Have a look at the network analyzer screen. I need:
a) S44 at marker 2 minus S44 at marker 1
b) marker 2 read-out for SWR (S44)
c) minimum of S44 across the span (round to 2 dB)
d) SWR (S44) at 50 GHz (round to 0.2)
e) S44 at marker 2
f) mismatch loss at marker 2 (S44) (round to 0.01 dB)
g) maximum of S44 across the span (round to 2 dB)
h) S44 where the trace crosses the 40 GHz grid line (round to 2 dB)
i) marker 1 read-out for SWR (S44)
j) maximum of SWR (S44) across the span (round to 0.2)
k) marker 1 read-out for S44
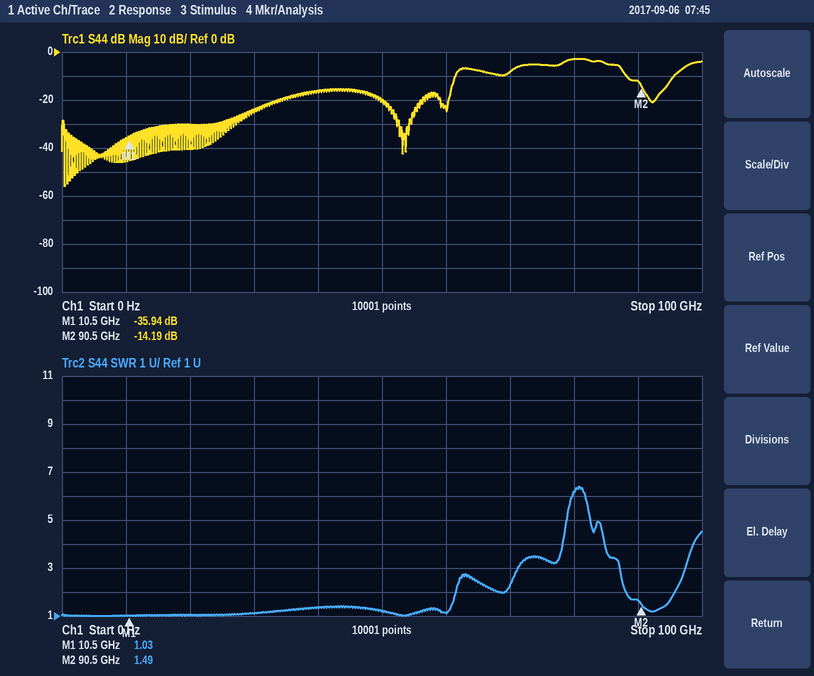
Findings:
21.75 dB
1.49
-56 dB
1.2
-14.19 dB
0.17 dB
-2 dB
-16 dB
1.03
6.4
-35.94 dB
